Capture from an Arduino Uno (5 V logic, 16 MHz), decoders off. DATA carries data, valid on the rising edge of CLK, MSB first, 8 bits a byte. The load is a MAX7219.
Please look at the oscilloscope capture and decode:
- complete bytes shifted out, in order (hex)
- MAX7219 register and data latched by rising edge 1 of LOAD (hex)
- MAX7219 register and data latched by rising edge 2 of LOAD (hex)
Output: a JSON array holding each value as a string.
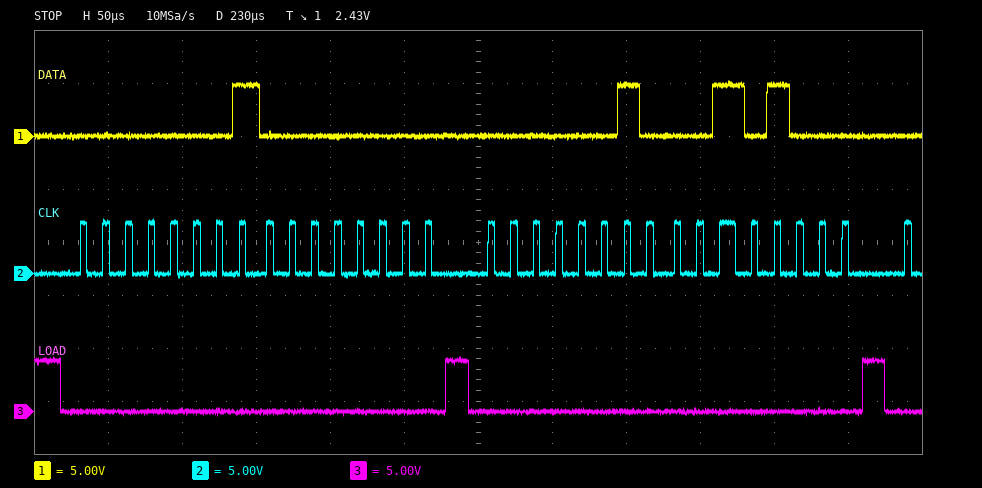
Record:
["01 00 02 28", "register 0x1, data 0x00", "register 0x2, data 0x28"]
